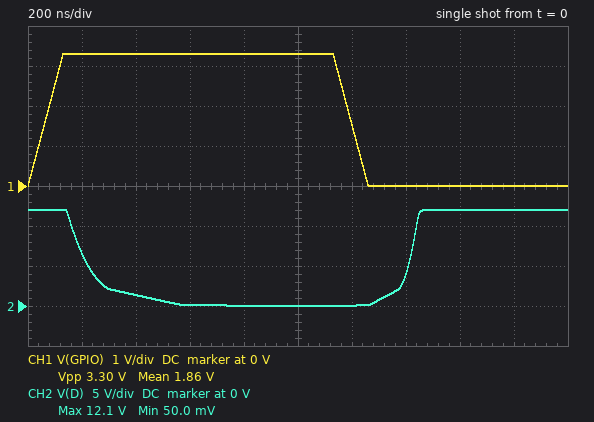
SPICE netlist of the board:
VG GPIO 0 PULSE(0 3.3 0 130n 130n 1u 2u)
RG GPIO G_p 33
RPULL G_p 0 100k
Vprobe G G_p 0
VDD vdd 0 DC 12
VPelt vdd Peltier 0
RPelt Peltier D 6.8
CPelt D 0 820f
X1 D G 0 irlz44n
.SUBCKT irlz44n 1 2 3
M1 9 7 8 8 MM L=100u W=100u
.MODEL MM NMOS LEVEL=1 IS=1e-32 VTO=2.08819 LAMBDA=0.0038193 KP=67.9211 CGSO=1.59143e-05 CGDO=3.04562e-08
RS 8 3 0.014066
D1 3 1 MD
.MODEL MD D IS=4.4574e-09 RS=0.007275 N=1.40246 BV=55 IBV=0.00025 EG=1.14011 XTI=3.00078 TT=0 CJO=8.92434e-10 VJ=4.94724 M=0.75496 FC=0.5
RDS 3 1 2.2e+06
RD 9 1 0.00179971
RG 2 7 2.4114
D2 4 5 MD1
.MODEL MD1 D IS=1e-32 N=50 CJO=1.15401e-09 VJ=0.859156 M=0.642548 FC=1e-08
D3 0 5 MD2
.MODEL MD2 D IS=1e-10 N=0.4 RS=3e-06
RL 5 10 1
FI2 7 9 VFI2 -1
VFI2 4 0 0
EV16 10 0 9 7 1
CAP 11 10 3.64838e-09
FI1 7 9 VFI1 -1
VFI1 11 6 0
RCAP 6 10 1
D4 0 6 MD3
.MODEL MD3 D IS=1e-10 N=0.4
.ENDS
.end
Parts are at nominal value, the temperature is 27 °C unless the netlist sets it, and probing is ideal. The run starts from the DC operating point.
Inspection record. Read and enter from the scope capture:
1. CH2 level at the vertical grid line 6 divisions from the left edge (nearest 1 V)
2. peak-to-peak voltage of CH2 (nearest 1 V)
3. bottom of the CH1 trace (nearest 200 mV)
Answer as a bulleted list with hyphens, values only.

- 0 V
- 12 V
- 0 V
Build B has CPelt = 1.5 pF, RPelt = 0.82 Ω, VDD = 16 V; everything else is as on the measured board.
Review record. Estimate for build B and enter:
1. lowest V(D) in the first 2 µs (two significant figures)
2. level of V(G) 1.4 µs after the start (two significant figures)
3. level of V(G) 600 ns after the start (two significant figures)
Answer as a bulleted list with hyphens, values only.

- 1.7 V
- 670 mV
- 3.0 V
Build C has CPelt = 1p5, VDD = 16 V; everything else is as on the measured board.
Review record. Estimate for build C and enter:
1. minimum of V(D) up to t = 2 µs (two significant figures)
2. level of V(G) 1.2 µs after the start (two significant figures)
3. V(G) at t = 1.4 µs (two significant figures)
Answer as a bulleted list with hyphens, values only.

- 69 mV
- 2.9 V
- 2.2 V
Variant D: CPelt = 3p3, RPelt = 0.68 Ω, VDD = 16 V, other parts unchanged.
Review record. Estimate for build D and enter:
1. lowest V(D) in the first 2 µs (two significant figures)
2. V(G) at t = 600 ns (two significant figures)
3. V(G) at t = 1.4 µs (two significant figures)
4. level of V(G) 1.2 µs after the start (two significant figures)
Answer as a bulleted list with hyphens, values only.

- 2.4 V
- 3.1 V
- 430 mV
- 3.0 V
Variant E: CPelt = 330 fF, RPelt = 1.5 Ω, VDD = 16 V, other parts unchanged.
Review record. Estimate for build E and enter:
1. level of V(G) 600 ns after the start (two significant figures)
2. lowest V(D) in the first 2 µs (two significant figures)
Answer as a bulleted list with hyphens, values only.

- 2.8 V
- 370 mV
